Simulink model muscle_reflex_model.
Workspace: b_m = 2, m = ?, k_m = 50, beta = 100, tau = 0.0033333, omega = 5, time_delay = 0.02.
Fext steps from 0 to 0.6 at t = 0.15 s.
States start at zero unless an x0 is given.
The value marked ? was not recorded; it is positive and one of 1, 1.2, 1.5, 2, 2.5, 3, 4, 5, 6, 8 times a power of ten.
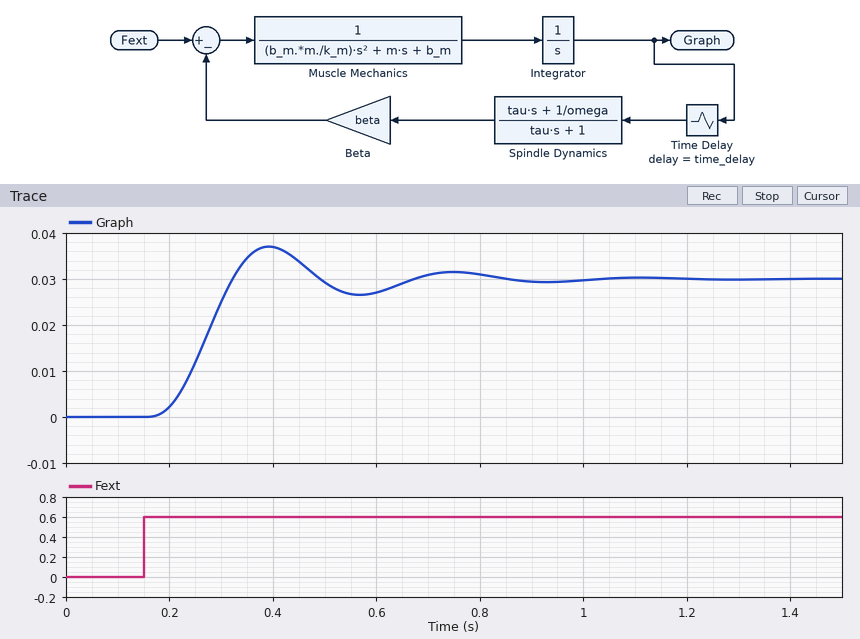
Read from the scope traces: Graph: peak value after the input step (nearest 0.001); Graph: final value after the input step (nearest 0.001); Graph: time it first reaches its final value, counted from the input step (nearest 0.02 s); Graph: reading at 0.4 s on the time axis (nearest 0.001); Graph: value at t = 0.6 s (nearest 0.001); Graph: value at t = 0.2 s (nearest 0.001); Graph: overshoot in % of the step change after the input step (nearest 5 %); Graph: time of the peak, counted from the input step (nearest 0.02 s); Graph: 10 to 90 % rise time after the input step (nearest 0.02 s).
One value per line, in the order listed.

0.037
0.030
0.18 s
0.037
0.027
0.002
25 %
0.24 s
0.10 s
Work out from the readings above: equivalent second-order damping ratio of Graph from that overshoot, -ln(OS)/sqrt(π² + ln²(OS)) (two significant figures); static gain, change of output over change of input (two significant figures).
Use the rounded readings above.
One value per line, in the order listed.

0.40
0.050
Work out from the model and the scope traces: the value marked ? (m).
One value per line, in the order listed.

0.1
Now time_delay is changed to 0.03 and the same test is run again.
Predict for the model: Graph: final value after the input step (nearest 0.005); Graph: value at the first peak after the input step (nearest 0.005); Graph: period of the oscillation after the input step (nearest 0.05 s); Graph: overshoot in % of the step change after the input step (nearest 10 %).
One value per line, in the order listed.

0.030
0.040
0.40 s
30 %
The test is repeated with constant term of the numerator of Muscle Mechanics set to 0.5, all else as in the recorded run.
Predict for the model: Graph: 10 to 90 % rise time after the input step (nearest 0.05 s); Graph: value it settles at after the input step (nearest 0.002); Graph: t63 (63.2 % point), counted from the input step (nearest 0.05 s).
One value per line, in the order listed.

0.25 s
0.030
0.20 s
